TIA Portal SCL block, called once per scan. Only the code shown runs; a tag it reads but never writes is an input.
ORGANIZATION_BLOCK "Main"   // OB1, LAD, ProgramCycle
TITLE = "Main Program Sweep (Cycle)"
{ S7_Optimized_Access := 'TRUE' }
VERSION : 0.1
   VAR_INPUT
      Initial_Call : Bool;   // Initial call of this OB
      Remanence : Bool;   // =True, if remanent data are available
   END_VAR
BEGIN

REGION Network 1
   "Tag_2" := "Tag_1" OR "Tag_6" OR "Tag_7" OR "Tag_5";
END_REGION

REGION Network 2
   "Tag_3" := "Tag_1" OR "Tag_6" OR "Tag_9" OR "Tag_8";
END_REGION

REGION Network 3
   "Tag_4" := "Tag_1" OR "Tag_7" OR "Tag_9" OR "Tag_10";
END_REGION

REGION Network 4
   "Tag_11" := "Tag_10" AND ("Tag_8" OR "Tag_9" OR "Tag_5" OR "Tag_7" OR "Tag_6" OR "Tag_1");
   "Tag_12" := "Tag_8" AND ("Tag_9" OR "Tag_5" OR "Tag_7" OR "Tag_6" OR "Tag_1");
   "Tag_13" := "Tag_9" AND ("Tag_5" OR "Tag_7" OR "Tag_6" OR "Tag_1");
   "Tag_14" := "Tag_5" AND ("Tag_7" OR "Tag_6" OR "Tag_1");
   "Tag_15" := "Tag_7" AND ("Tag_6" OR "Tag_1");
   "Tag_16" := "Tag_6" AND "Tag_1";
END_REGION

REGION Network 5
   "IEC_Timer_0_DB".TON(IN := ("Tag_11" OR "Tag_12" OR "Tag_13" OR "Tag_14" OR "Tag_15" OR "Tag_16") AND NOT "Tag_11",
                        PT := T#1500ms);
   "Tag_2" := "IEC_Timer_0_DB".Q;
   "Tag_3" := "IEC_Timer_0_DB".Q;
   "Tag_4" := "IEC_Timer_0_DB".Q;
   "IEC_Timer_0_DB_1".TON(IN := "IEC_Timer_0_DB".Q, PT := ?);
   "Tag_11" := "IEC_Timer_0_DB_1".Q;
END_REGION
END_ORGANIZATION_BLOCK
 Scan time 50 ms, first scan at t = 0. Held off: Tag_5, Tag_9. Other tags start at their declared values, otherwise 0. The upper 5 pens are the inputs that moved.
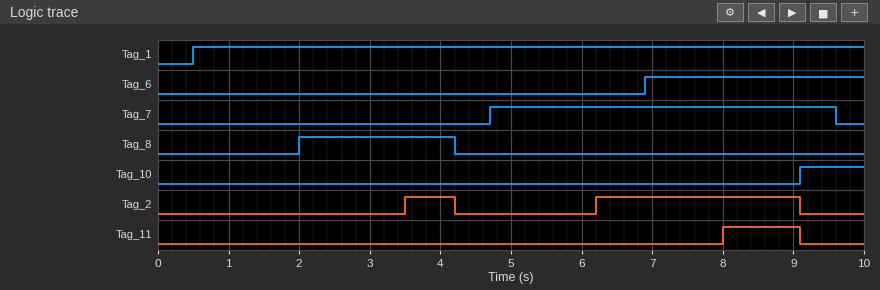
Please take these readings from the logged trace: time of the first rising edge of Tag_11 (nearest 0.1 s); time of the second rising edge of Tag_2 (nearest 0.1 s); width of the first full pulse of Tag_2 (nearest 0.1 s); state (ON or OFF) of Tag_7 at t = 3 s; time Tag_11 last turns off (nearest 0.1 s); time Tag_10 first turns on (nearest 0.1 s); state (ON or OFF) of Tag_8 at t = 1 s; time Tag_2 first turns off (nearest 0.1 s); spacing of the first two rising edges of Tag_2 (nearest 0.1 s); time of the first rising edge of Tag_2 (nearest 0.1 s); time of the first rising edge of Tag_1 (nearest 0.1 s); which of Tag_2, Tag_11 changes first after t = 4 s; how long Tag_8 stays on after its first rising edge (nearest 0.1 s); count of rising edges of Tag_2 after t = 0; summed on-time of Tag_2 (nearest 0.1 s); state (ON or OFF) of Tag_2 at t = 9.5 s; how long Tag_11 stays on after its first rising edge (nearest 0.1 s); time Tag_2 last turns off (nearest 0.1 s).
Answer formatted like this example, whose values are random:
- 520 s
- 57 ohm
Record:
- 8.0 s
- 6.2 s
- 0.7 s
- OFF
- 9.1 s
- 9.1 s
- OFF
- 4.2 s
- 2.7 s
- 3.5 s
- 0.5 s
- Tag_2
- 2.2 s
- 2
- 3.6 s
- OFF
- 1.1 s
- 9.1 s
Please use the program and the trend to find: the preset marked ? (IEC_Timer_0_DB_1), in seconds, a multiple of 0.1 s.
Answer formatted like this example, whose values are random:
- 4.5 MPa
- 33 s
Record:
- 1.8 s
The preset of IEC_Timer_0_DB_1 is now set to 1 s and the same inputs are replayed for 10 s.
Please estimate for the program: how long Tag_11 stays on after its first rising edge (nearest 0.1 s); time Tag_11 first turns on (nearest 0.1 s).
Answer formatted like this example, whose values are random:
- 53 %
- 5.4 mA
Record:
- 1.9 s
- 7.2 s
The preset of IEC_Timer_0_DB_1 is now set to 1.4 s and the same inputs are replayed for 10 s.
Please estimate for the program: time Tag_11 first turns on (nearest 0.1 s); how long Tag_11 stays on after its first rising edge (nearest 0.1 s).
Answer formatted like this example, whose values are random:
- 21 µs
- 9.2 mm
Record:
- 7.6 s
- 1.5 s
